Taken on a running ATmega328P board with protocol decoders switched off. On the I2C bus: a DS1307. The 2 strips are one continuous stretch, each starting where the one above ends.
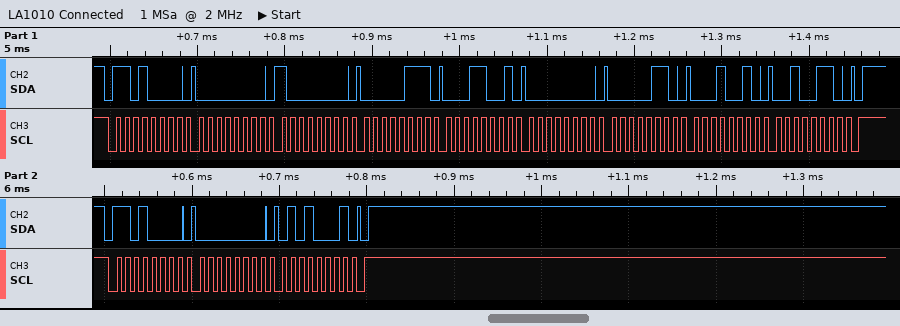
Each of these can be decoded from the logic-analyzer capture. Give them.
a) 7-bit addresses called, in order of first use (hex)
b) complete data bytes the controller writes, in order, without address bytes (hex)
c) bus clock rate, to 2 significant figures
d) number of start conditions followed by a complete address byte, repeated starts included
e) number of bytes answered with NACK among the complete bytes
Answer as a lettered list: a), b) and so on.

a) 0x68
b) 00 80 07 19 00 06 12 26 00 51
c) 100 kHz
d) 2
e) 0
